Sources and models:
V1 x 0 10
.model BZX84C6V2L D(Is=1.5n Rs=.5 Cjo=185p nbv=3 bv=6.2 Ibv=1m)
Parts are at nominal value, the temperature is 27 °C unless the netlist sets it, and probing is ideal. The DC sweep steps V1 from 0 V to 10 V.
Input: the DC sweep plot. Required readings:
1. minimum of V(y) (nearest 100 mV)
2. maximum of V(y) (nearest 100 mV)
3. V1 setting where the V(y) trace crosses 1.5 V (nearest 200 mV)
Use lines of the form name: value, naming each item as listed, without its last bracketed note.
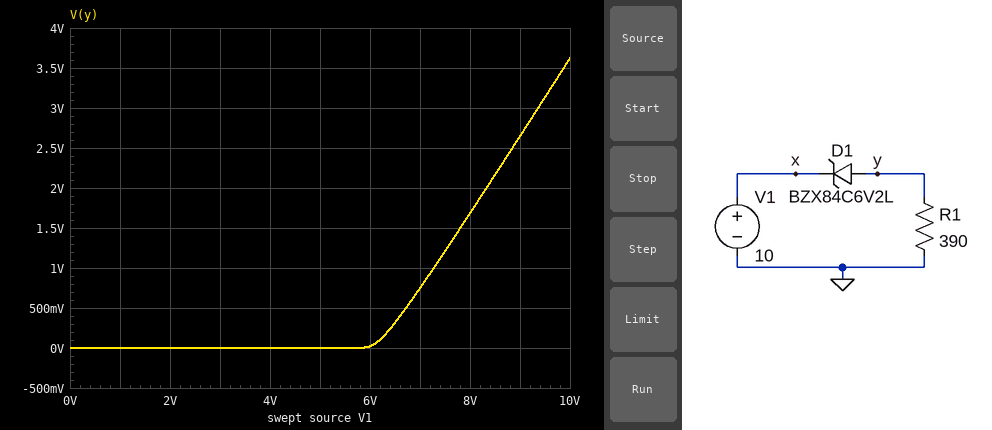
minimum of V(y): 0 V
maximum of V(y): 3.6 V
V1 setting where the V(y) trace crosses 1.5 V: 7.8 V
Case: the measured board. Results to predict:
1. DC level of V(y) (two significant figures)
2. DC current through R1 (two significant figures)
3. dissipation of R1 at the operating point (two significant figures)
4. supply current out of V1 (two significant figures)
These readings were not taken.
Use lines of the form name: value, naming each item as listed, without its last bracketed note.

DC level of V(y): 3.6 V
DC current through R1: 9.3 mA
dissipation of R1 at the operating point: 34 mW
supply current out of V1: 9.3 mA
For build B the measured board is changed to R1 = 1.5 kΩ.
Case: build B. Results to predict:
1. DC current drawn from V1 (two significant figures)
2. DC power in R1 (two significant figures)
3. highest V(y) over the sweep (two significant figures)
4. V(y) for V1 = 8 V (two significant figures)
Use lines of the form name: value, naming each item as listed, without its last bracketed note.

DC current drawn from V1: 2.5 mA
DC power in R1: 9.3 mW
highest V(y) over the sweep: 3.7 V
V(y) for V1 = 8 V: 1.8 V
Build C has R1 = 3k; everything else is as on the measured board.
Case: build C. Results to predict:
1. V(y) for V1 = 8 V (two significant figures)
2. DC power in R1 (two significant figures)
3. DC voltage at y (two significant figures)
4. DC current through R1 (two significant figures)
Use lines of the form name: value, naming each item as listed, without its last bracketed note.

V(y) for V1 = 8 V: 1.8 V
DC power in R1: 4.8 mW
DC voltage at y: 3.8 V
DC current through R1: 1.3 mA
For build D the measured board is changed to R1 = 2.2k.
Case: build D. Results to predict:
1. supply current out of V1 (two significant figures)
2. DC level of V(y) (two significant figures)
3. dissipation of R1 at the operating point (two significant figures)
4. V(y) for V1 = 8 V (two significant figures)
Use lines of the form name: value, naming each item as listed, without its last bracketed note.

supply current out of V1: 1.7 mA
DC level of V(y): 3.8 V
dissipation of R1 at the operating point: 6.4 mW
V(y) for V1 = 8 V: 1.8 V
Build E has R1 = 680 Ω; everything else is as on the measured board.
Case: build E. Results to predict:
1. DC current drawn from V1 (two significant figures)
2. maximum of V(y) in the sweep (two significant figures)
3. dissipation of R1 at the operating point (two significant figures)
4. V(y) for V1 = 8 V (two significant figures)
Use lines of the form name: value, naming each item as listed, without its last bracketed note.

DC current drawn from V1: 5.4 mA
maximum of V(y) in the sweep: 3.7 V
dissipation of R1 at the operating point: 20 mW
V(y) for V1 = 8 V: 1.7 V
